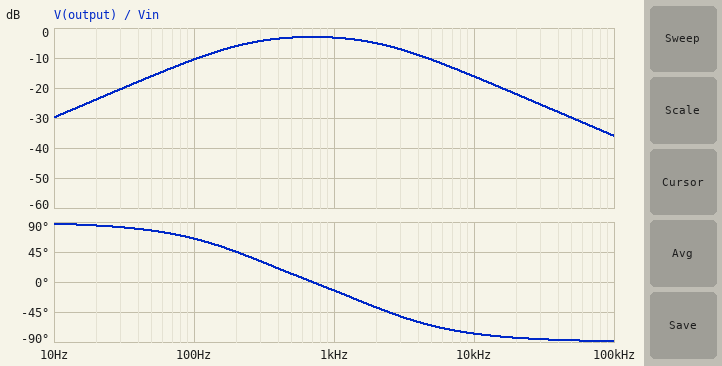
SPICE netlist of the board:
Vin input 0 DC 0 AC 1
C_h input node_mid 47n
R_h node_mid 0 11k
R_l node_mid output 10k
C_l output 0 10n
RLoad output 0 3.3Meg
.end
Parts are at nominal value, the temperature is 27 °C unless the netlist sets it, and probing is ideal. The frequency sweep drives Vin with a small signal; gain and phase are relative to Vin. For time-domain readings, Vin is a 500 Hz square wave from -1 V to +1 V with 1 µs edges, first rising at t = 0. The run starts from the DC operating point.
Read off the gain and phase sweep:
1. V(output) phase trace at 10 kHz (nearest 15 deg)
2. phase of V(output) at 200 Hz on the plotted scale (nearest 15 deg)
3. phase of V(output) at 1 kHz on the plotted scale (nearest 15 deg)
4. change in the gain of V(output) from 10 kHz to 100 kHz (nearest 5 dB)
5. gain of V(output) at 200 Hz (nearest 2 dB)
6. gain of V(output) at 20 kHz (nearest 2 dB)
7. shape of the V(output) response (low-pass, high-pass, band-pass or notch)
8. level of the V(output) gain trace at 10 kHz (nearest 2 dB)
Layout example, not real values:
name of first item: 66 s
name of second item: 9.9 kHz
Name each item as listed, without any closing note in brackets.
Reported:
V(output) phase trace at 10 kHz: -75 deg
phase of V(output) at 200 Hz on the plotted scale: 45 deg
phase of V(output) at 1 kHz on the plotted scale: -15 deg
change in the gain of V(output) from 10 kHz to 100 kHz: -20 dB
gain of V(output) at 200 Hz: -6 dB
gain of V(output) at 20 kHz: -22 dB
shape of the V(output) response: band-pass
level of the V(output) gain trace at 10 kHz: -16 dB
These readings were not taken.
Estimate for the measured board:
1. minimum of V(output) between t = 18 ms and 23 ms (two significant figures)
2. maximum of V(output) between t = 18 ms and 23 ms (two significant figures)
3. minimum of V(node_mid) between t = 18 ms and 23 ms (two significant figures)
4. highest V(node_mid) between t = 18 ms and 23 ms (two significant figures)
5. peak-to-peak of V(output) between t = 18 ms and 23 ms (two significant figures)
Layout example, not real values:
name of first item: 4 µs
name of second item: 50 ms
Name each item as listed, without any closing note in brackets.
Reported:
minimum of V(output) between t = 18 ms and 23 ms: -950 mV
maximum of V(output) between t = 18 ms and 23 ms: 950 mV
minimum of V(node_mid) between t = 18 ms and 23 ms: -1.7 V
highest V(node_mid) between t = 18 ms and 23 ms: 1.7 V
peak-to-peak of V(output) between t = 18 ms and 23 ms: 1.9 V
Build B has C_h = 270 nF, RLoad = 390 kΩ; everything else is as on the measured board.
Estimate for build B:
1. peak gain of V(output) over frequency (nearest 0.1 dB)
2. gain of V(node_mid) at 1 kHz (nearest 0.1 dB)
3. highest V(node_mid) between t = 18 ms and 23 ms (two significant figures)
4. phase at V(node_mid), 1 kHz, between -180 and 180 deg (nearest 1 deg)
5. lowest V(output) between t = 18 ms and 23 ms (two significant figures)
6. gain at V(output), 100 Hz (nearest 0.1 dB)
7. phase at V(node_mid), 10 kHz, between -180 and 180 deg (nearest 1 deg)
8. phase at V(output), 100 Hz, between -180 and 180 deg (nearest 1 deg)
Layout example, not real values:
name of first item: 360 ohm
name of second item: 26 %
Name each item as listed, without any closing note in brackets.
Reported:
peak gain of V(output) over frequency: -0.8 dB
gain of V(node_mid) at 1 kHz: -0.2 dB
highest V(node_mid) between t = 18 ms and 23 ms: 1.2 V
phase at V(node_mid), 1 kHz, between -180 and 180 deg: 4 deg
lowest V(output) between t = 18 ms and 23 ms: -960 mV
gain at V(output), 100 Hz: -1.6 dB
phase at V(node_mid), 10 kHz, between -180 and 180 deg: 1 deg
phase at V(output), 100 Hz, between -180 and 180 deg: 25 deg
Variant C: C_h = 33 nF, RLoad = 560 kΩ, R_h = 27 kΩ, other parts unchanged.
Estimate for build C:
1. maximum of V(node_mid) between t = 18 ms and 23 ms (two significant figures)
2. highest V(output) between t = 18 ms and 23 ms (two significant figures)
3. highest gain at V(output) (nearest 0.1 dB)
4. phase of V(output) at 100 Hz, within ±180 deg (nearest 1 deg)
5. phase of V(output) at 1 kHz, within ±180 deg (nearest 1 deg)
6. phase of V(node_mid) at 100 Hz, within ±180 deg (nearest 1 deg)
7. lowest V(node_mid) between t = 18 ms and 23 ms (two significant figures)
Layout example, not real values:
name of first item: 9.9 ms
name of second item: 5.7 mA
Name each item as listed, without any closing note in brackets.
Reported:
maximum of V(node_mid) between t = 18 ms and 23 ms: 1.6 V
highest V(output) between t = 18 ms and 23 ms: 850 mV
highest gain at V(output): -3.1 dB
phase of V(output) at 100 Hz, within ±180 deg: 52 deg
phase of V(output) at 1 kHz, within ±180 deg: -17 deg
phase of V(node_mid) at 100 Hz, within ±180 deg: 56 deg
lowest V(node_mid) between t = 18 ms and 23 ms: -1.6 V
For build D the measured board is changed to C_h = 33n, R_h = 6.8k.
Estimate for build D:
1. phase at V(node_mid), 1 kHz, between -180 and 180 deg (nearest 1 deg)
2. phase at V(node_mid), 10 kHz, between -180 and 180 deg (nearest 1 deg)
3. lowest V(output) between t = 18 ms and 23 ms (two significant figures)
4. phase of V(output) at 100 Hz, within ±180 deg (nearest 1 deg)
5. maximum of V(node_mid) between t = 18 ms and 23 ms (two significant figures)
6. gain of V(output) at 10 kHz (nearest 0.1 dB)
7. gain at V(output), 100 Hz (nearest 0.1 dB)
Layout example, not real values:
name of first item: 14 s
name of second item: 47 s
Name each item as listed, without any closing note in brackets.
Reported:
phase at V(node_mid), 1 kHz, between -180 and 180 deg: 35 deg
phase at V(node_mid), 10 kHz, between -180 and 180 deg: 7 deg
lowest V(output) between t = 18 ms and 23 ms: -860 mV
phase of V(output) at 100 Hz, within ±180 deg: 76 deg
maximum of V(node_mid) between t = 18 ms and 23 ms: 1.9 V
gain of V(output) at 10 kHz: -16.2 dB
gain at V(output), 100 Hz: -17.2 dB
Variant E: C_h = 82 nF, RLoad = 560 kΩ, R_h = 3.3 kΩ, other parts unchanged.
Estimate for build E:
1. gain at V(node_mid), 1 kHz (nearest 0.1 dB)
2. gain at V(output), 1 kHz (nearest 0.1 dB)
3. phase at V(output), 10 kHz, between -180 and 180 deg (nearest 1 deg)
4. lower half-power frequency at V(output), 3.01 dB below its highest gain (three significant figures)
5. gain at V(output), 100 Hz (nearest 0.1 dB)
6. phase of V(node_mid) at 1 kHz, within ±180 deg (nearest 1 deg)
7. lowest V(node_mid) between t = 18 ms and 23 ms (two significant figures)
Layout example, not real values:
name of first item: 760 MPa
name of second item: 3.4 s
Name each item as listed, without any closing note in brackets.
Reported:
gain at V(node_mid), 1 kHz: -2.0 dB
gain at V(output), 1 kHz: -3.6 dB
phase at V(output), 10 kHz, between -180 and 180 deg: -76 deg
lower half-power frequency at V(output), 3.01 dB below its highest gain: 348 Hz
gain at V(output), 100 Hz: -15.8 dB
phase of V(node_mid) at 1 kHz, within ±180 deg: 31 deg
lowest V(node_mid) between t = 18 ms and 23 ms: -1.9 V
